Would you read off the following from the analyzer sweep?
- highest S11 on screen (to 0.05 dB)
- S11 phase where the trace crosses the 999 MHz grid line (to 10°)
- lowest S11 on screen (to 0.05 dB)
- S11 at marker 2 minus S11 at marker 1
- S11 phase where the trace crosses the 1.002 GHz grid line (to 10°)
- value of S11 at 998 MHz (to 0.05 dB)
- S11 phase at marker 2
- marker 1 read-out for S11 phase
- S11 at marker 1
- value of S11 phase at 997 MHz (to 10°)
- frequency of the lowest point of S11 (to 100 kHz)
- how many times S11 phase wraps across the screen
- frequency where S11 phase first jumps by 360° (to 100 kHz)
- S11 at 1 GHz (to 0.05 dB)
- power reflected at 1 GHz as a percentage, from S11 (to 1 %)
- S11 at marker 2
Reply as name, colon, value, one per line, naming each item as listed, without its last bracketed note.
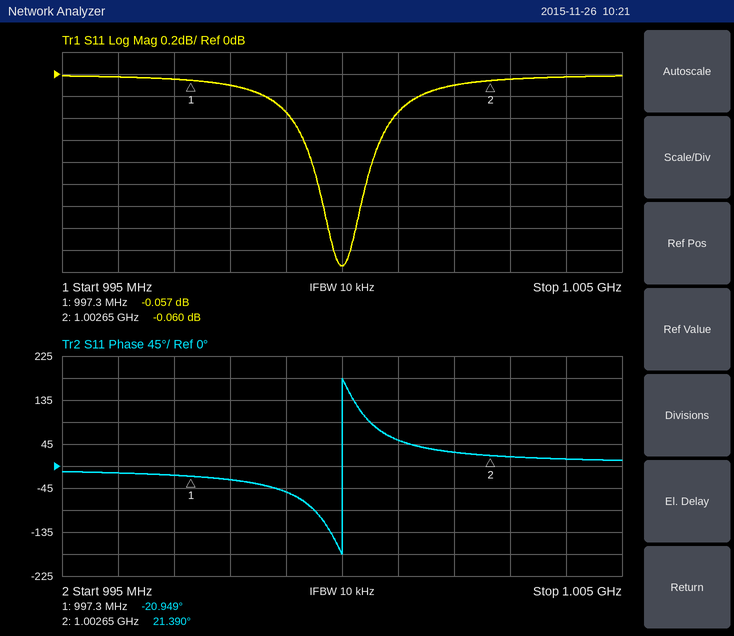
highest S11 on screen: 0.00 dB
S11 phase where the trace crosses the 999 MHz grid line: -50°
lowest S11 on screen: -1.75 dB
S11 at marker 2 minus S11 at marker 1: -0.003 dB
S11 phase where the trace crosses the 1.002 GHz grid line: 30°
value of S11 at 998 MHz: -0.10 dB
S11 phase at marker 2: 21.390°
marker 1 read-out for S11 phase: -20.949°
S11 at marker 1: -0.057 dB
value of S11 phase at 997 MHz: -20°
frequency of the lowest point of S11: 1.0000 GHz
how many times S11 phase wraps across the screen: 1
frequency where S11 phase first jumps by 360°: 1.0000 GHz
S11 at 1 GHz: -1.75 dB
power reflected at 1 GHz as a percentage, from S11: 67 %
S11 at marker 2: -0.060 dB
